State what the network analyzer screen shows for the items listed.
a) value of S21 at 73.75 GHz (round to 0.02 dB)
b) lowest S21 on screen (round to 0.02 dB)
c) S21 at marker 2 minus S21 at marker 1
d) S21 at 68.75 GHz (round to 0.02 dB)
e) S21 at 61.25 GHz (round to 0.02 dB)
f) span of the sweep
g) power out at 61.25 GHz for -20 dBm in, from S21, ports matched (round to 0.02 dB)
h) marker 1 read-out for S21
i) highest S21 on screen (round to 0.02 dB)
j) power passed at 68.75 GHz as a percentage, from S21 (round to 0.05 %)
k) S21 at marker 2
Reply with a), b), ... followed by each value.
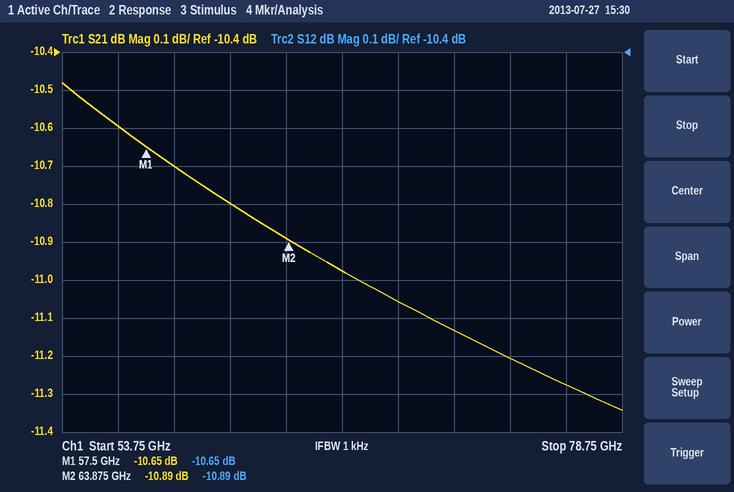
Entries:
a) -11.20 dB
b) -11.34 dB
c) -0.24 dB
d) -11.06 dB
e) -10.80 dB
f) 25 GHz
g) -30.80 dBm
h) -10.65 dB
i) -10.48 dB
j) 7.85 %
k) -10.89 dB
